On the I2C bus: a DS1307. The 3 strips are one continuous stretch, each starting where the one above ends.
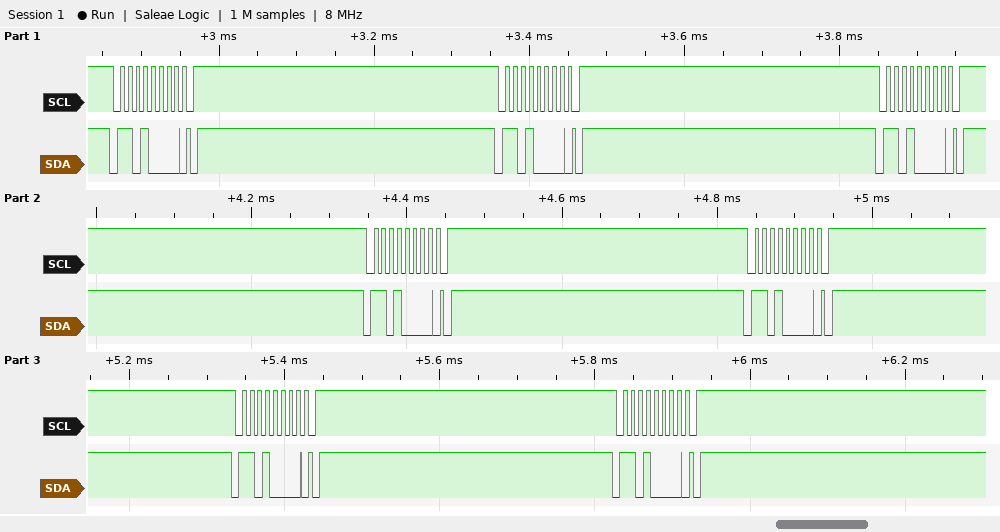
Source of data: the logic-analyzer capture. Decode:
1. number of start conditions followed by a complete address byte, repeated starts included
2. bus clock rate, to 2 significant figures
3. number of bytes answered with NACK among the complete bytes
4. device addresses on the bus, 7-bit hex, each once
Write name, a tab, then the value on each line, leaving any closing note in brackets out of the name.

number of start conditions followed by a complete address byte, repeated starts included	7
bus clock rate, to 2 significant figures	100 kHz
number of bytes answered with NACK among the complete bytes	0
device addresses on the bus, 7-bit hex, each once	0x68
